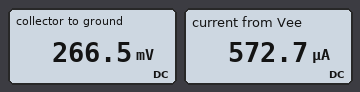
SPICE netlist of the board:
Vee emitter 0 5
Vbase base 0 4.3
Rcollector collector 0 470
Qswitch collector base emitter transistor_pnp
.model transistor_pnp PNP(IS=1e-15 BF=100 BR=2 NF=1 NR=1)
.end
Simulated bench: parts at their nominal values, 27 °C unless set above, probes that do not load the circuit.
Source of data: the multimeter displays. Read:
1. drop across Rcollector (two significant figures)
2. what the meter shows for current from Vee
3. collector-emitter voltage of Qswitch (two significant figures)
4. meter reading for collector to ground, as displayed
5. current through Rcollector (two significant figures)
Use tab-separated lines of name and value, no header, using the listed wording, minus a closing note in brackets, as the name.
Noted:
drop across Rcollector	270 mV
what the meter shows for current from Vee	572.7 µA
collector-emitter voltage of Qswitch	-4.7 V
meter reading for collector to ground, as displayed	266.5 mV
current through Rcollector	570 µA
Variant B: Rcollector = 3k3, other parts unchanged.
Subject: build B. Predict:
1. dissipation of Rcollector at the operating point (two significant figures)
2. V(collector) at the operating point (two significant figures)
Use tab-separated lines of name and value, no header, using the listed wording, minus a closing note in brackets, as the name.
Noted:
dissipation of Rcollector at the operating point	1.1 mW
V(collector) at the operating point	1.9 V
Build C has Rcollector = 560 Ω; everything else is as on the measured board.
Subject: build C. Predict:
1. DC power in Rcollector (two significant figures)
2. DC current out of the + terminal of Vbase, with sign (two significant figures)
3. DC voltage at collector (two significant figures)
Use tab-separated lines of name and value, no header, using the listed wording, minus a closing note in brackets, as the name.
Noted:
DC power in Rcollector	180 µW
DC current out of the + terminal of Vbase, with sign	-5.7 µA
DC voltage at collector	320 mV
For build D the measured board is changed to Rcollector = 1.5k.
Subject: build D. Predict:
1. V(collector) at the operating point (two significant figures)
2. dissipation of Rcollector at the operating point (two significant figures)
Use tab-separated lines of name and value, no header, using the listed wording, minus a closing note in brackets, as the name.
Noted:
V(collector) at the operating point	850 mV
dissipation of Rcollector at the operating point	480 µW
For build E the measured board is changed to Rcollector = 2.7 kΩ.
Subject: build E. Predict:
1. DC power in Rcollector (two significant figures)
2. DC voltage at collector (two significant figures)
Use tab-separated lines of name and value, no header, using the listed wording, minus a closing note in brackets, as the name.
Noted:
DC power in Rcollector	870 µW
DC voltage at collector	1.5 V
